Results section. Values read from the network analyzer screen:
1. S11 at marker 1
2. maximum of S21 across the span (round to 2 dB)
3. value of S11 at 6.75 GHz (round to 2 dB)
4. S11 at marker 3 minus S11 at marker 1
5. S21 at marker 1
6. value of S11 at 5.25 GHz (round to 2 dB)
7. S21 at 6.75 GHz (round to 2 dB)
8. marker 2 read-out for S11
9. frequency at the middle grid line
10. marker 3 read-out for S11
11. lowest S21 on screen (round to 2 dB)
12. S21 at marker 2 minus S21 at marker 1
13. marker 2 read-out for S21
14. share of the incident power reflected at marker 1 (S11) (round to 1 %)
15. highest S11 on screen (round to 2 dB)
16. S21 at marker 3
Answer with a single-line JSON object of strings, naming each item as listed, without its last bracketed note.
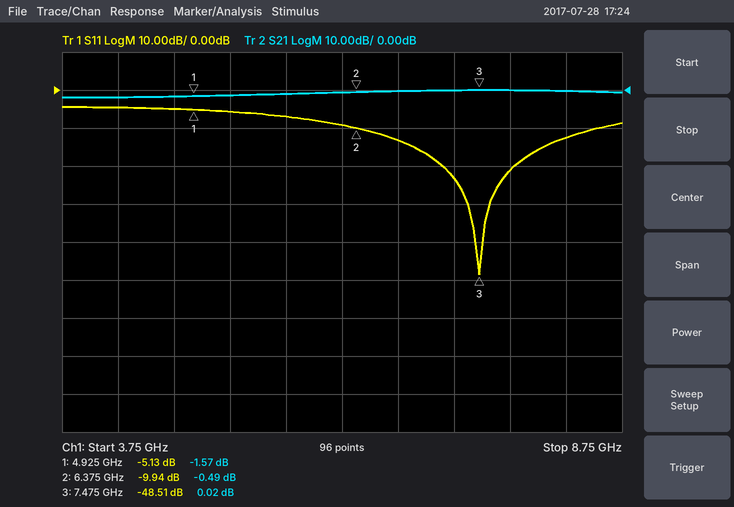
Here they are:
{"S11 at marker 1": "-5.13 dB", "maximum of S21 across the span": "0 dB", "value of S11 at 6.75 GHz": "-14 dB", "S11 at marker 3 minus S11 at marker 1": "-43.38 dB", "S21 at marker 1": "-1.57 dB", "value of S11 at 5.25 GHz": "-6 dB", "S21 at 6.75 GHz": "0 dB", "marker 2 read-out for S11": "-9.94 dB", "frequency at the middle grid line": "6.25 GHz", "marker 3 read-out for S11": "-48.51 dB", "lowest S21 on screen": "-2 dB", "S21 at marker 2 minus S21 at marker 1": "1.08 dB", "marker 2 read-out for S21": "-0.49 dB", "share of the incident power reflected at marker 1 (S11)": "31 %", "highest S11 on screen": "-4 dB", "S21 at marker 3": "0.02 dB"}
